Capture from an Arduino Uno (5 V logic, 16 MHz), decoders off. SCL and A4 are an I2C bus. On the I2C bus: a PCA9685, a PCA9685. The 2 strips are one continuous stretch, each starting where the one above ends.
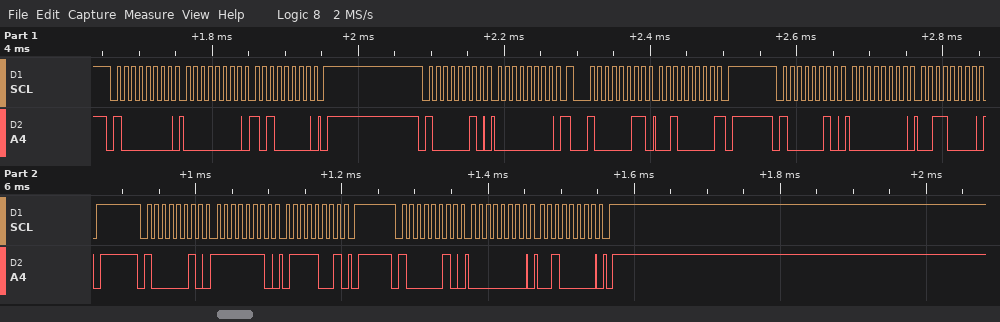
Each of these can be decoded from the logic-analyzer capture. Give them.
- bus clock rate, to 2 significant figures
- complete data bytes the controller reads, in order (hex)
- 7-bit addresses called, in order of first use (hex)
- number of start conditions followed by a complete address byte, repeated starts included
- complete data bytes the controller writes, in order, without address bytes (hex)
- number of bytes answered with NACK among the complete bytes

100 kHz
20
0x40 0x41
6
00 A0 00 00 30 FE 79 00 20
1
